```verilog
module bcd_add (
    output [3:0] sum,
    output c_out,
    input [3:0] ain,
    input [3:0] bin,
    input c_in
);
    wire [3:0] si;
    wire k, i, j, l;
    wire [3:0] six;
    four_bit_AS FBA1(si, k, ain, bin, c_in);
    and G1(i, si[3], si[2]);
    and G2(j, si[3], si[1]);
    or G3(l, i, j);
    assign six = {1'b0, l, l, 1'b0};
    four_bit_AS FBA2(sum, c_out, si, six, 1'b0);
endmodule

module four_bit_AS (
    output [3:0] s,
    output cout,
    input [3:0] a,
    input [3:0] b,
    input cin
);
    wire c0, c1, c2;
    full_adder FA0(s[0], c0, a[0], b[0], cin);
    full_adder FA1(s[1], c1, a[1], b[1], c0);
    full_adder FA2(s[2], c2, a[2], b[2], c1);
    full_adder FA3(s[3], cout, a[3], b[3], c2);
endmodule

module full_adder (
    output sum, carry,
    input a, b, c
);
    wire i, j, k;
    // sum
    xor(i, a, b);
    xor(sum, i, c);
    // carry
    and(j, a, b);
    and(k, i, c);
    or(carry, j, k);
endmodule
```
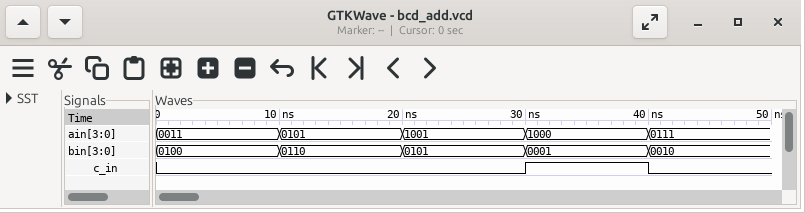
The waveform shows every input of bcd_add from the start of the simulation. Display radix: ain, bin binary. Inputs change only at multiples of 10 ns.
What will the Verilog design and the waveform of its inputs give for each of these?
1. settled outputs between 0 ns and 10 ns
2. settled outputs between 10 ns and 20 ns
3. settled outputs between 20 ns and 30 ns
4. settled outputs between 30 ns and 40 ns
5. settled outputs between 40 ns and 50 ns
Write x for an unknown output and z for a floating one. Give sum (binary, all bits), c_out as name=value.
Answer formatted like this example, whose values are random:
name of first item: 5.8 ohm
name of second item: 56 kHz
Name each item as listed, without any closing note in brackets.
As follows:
settled outputs between 0 ns and 10 ns: sum=0111, c_out=0
settled outputs between 10 ns and 20 ns: sum=0001, c_out=1
settled outputs between 20 ns and 30 ns: sum=0100, c_out=1
settled outputs between 30 ns and 40 ns: sum=0000, c_out=1
settled outputs between 40 ns and 50 ns: sum=1001, c_out=0
